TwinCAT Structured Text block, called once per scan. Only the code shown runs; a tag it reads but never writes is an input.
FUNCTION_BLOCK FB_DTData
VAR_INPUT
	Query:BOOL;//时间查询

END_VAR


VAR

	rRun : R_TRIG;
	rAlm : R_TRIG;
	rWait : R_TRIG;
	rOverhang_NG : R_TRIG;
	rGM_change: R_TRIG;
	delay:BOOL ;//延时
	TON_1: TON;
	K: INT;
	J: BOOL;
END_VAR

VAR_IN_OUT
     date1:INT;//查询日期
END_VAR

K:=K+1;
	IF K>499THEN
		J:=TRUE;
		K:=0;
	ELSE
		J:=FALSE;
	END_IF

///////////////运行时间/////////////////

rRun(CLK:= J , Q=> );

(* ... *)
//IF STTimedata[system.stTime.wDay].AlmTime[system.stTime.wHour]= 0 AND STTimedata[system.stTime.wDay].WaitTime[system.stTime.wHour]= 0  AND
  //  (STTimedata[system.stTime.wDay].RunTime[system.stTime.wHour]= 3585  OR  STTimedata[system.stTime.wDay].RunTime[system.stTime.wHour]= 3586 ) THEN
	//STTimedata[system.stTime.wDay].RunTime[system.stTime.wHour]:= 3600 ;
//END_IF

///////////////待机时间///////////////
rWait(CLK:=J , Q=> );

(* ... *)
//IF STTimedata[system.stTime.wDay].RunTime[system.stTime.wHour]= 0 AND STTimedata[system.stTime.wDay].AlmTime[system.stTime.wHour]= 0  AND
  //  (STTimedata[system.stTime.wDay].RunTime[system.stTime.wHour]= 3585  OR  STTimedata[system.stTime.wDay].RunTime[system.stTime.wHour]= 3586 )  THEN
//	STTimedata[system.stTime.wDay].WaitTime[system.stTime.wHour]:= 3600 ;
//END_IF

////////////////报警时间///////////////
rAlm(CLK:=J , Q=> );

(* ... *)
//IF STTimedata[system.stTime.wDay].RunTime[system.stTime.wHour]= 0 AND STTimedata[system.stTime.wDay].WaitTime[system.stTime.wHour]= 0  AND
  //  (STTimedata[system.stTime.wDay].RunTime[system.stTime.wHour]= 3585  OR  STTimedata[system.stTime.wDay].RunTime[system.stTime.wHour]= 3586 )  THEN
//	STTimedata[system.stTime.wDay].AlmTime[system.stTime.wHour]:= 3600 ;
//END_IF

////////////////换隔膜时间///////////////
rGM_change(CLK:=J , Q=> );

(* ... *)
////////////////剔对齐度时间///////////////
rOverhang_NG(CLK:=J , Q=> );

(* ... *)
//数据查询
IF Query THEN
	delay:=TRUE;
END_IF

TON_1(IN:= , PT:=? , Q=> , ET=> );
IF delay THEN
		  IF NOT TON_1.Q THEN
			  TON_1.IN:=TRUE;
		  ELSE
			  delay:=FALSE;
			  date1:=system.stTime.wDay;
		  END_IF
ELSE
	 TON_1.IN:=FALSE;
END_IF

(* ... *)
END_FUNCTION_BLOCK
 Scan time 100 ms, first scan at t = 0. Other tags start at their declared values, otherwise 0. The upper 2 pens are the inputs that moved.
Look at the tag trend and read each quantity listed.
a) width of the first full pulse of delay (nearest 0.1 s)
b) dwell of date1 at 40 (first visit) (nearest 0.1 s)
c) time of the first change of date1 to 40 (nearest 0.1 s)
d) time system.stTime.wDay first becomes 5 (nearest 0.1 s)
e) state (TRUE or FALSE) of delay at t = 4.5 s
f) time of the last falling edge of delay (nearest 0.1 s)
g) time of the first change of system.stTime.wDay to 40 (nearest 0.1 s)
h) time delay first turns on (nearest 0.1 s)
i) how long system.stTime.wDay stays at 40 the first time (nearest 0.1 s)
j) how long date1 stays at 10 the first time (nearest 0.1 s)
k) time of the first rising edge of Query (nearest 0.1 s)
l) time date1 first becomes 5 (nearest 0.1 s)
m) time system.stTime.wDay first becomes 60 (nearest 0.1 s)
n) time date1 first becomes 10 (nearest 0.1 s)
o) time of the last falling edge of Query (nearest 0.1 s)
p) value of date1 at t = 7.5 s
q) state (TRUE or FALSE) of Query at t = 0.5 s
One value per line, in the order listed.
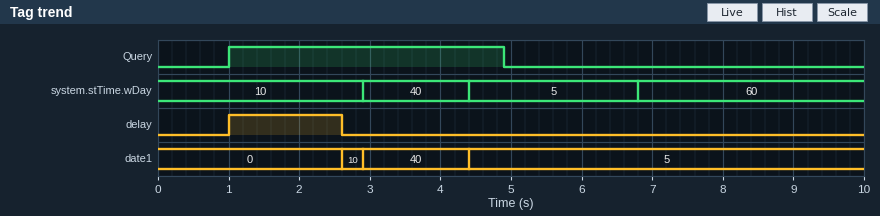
1.6 s
1.5 s
2.9 s
4.4 s
FALSE
2.6 s
2.9 s
1.0 s
1.5 s
0.3 s
1.0 s
4.4 s
6.8 s
2.6 s
4.9 s
5
FALSE
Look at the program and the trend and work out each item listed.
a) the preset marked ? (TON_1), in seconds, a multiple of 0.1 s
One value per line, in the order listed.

1.5 s
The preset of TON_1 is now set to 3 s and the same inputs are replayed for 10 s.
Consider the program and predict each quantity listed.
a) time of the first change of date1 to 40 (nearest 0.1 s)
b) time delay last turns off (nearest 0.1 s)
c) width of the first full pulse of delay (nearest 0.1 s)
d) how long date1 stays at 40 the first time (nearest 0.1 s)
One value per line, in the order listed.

4.1 s
4.1 s
3.1 s
0.3 s
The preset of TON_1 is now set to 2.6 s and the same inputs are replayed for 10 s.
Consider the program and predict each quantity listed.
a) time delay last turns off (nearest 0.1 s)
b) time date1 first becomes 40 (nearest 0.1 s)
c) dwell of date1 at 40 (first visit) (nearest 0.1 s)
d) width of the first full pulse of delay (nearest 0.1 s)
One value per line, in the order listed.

3.7 s
3.7 s
0.7 s
2.7 s
